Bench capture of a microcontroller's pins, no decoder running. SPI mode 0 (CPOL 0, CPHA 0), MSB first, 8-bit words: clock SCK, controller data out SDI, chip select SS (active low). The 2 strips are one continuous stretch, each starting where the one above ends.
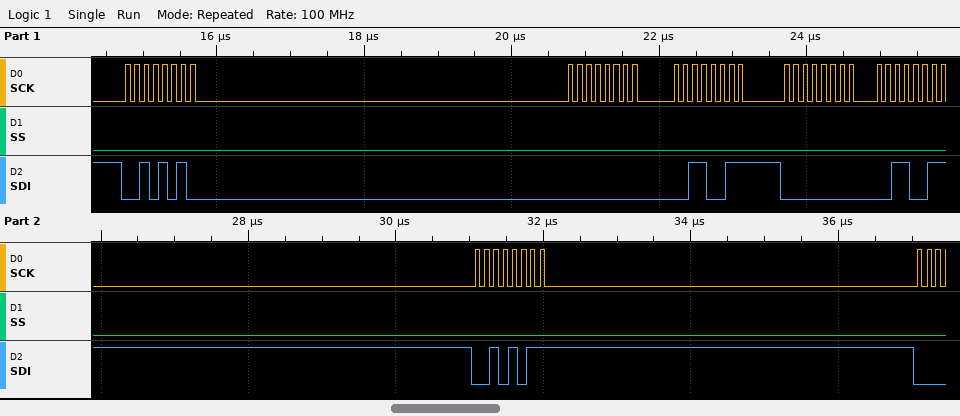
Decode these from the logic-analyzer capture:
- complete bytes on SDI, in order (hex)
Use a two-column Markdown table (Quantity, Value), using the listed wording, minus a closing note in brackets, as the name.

| Quantity | Value |
|---|---|
| complete bytes on SDI, in order | 2A 00 33 00 33 2B |
